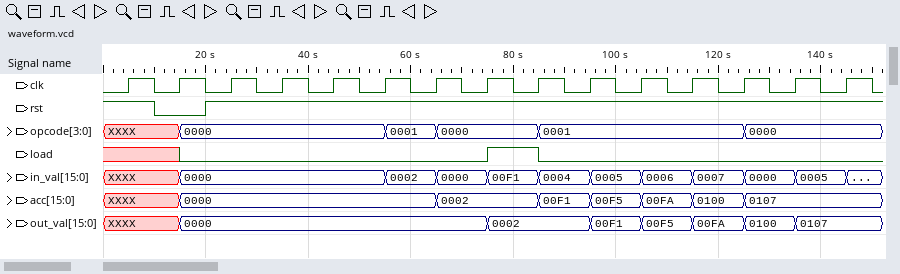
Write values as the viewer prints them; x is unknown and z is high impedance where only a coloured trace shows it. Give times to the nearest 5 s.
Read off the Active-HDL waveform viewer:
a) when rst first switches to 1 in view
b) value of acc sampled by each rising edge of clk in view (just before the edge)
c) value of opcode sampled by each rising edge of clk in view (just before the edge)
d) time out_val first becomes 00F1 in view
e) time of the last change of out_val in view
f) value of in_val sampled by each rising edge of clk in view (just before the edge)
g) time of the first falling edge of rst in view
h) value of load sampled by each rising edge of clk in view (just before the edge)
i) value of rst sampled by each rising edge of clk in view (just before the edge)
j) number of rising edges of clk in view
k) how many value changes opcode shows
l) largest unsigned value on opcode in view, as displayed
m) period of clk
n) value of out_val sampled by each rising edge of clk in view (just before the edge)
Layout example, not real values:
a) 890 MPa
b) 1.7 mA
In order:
a) 20 s
b) XXXX, XXXX, 0000, 0000, 0000, 0000, 0000, 0002, 0002, 00F1, 00F5, 00FA, 0100, 0107, 0107
c) XXXX, XXXX, 0000, 0000, 0000, 0000, 0001, 0000, 0000, 0001, 0001, 0001, 0001, 0000, 0000
d) 95 s
e) 135 s
f) XXXX, XXXX, 0000, 0000, 0000, 0000, 0002, 0000, 00F1, 0004, 0005, 0006, 0007, 0000, 0005
g) 10 s
h) x x 0 0 0 0 0 0 1 0 0 0 0 0 0
i) 1 0 1 1 1 1 1 1 1 1 1 1 1 1 1
j) 15
k) 5
l) 0001
m) 10 s
n) XXXX, XXXX, 0000, 0000, 0000, 0000, 0000, 0000, 0002, 0002, 00F1, 00F5, 00FA, 0100, 0107
